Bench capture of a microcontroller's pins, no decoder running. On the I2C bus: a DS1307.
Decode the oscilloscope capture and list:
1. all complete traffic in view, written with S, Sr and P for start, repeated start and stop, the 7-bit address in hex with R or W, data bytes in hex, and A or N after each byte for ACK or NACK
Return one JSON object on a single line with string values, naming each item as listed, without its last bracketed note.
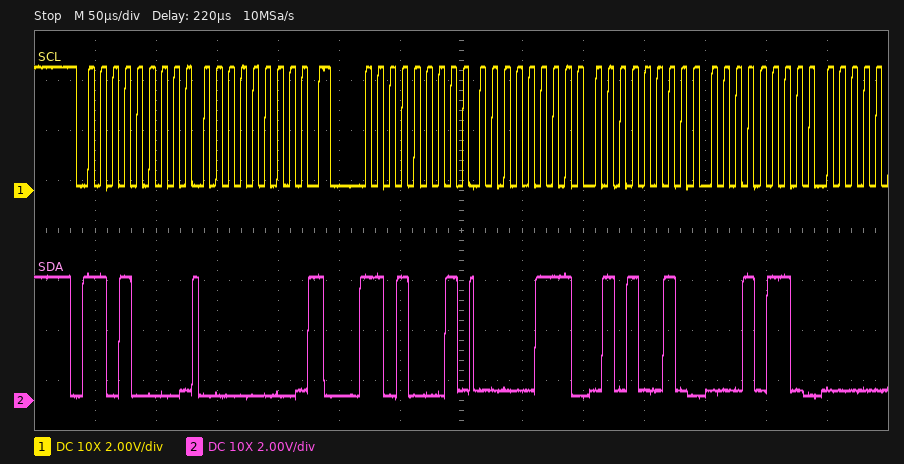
{"all complete traffic in view, written with S, Sr and P for start, repeated start and stop, the 7-bit address in hex with R or W, data bytes in hex, and A or N after each byte for ACK or NACK": "S 68W A 00 A Sr 68R A 07 A 52 A 16 A"}
